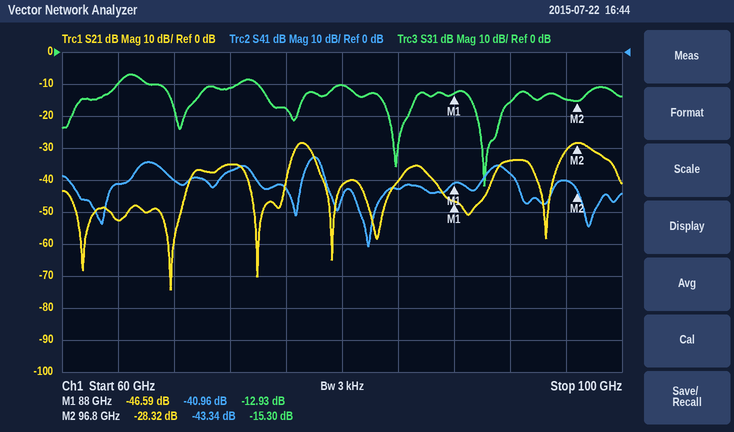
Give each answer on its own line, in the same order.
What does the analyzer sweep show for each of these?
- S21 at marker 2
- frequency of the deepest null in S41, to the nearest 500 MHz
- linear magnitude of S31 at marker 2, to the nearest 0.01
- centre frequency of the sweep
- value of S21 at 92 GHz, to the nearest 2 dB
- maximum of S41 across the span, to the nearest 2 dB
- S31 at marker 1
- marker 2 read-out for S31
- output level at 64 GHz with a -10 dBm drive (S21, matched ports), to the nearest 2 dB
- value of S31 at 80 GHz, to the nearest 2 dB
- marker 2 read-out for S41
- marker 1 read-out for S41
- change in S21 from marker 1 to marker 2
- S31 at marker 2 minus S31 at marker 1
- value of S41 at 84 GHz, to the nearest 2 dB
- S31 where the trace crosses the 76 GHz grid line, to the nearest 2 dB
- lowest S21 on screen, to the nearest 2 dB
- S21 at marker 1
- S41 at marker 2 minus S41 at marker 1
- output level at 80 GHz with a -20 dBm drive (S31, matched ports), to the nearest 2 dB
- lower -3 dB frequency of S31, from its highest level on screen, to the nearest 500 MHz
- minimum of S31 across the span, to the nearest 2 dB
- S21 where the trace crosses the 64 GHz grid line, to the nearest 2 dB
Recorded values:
-28.32 dB
82.0 GHz
0.17
80 GHz
-34 dB
-32 dB
-12.93 dB
-15.30 dB
-62 dBm
-10 dB
-43.34 dB
-40.96 dB
18.27 dB
-2.37 dB
-42 dB
-18 dB
-74 dB
-46.59 dB
-2.38 dB
-30 dBm
64.0 GHz
-42 dB
-52 dB
